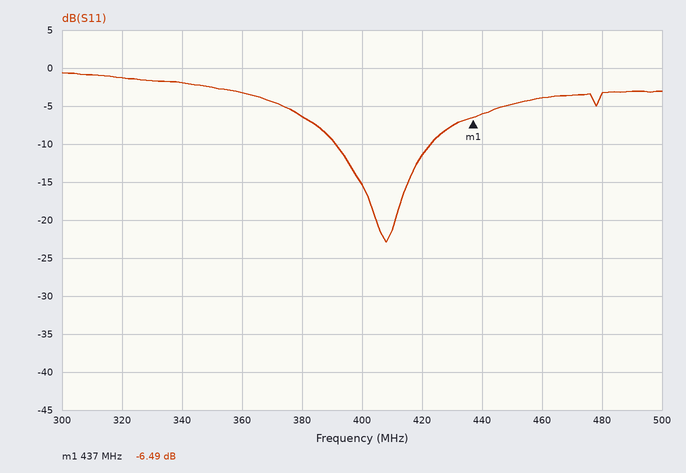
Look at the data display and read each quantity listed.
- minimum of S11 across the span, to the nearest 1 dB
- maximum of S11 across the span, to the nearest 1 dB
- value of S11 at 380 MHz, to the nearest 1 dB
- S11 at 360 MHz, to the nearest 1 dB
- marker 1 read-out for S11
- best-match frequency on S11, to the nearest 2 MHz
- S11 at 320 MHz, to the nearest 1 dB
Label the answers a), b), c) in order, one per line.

a) -23 dB
b) -1 dB
c) -6 dB
d) -3 dB
e) -6.49 dB
f) 408 MHz
g) -1 dB
